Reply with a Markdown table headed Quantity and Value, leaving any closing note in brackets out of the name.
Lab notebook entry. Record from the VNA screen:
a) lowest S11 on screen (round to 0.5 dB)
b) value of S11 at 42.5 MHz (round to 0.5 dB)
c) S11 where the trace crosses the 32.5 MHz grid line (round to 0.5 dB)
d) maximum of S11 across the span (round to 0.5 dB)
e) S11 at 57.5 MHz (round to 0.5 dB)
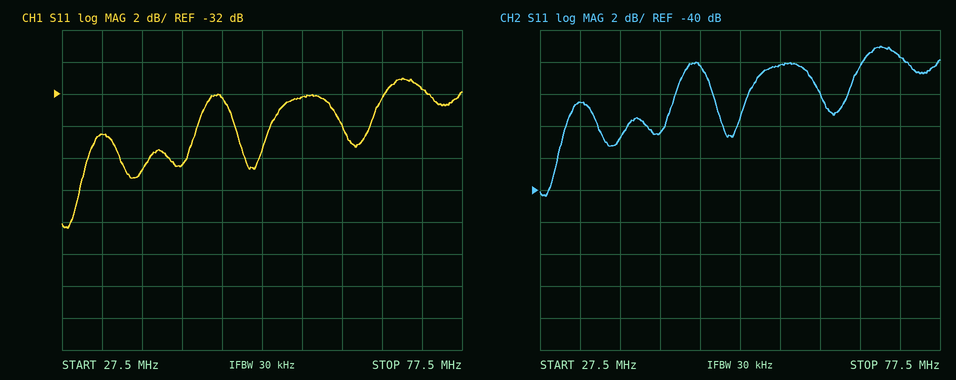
| Quantity | Value |
|---|---|
| lowest S11 on screen | -40.5 dB |
| value of S11 at 42.5 MHz | -36.5 dB |
| S11 where the trace crosses the 32.5 MHz grid line | -34.5 dB |
| maximum of S11 across the span | -31.0 dB |
| S11 at 57.5 MHz | -32.0 dB |
